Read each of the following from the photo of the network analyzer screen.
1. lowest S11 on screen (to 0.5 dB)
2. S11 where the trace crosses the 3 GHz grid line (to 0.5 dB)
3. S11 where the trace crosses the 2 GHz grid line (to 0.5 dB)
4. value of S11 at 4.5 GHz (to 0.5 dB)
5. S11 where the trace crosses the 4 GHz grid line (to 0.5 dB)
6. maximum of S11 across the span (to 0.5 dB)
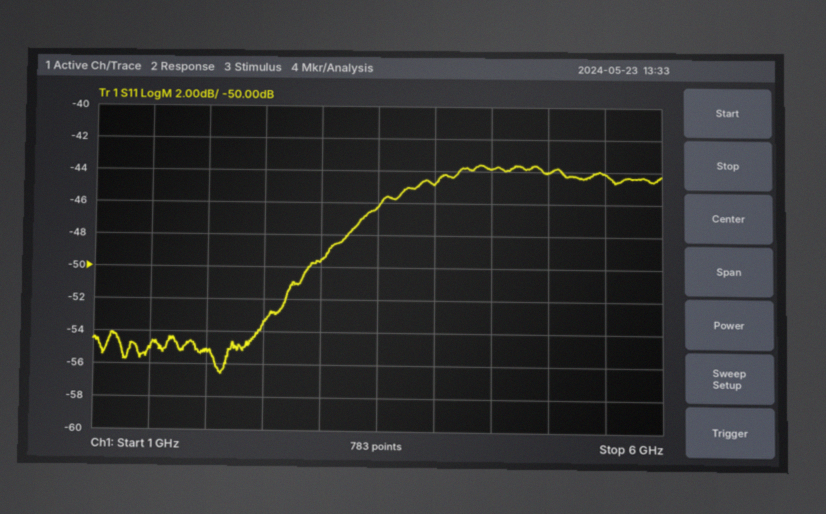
-56.5 dB
-49.5 dB
-55.0 dB
-44.0 dB
-45.0 dB
-43.5 dB
